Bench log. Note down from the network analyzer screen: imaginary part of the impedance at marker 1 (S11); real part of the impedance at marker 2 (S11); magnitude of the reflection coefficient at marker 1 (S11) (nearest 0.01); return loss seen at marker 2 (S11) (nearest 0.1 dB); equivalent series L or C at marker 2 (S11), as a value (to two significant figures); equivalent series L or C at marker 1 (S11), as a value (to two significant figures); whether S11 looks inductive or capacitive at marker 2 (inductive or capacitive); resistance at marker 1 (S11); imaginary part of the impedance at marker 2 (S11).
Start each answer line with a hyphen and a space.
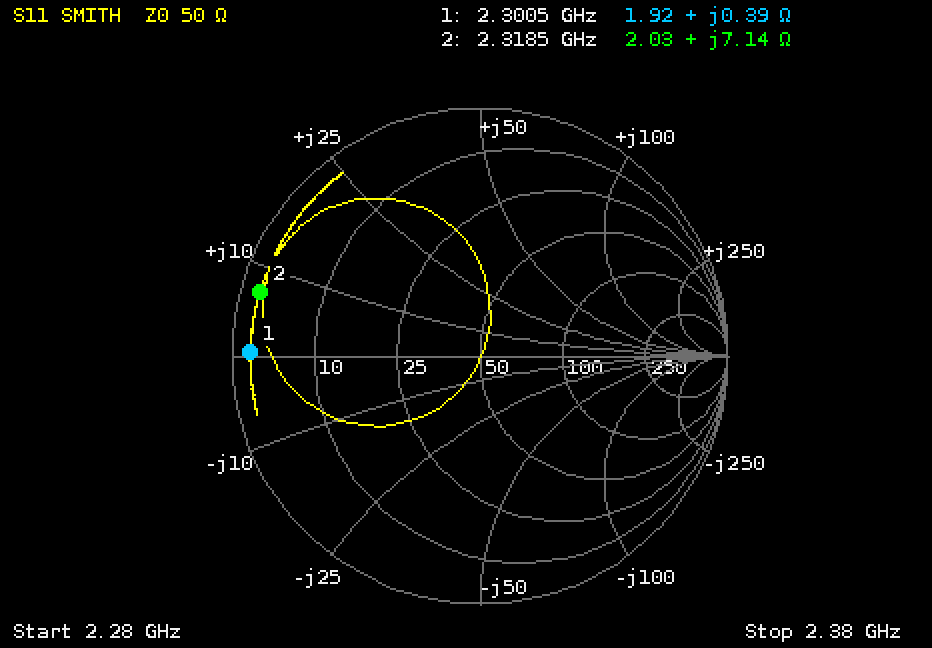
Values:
- +0.39 Ω
- 2.03 Ω
- 0.93
- 0.7 dB
- 490 pH
- 27 pH
- inductive
- 1.92 Ω
- +7.14 Ω
